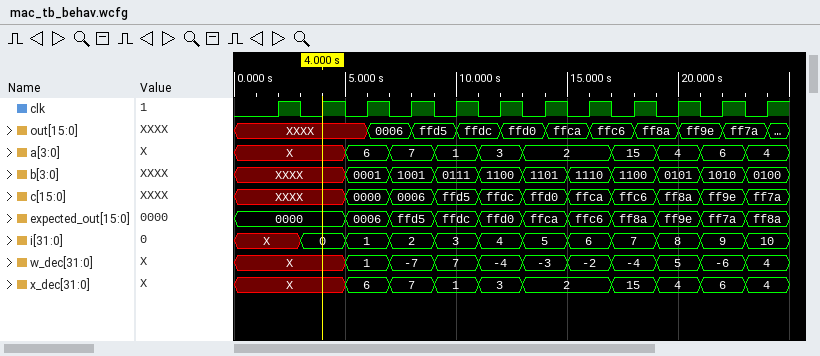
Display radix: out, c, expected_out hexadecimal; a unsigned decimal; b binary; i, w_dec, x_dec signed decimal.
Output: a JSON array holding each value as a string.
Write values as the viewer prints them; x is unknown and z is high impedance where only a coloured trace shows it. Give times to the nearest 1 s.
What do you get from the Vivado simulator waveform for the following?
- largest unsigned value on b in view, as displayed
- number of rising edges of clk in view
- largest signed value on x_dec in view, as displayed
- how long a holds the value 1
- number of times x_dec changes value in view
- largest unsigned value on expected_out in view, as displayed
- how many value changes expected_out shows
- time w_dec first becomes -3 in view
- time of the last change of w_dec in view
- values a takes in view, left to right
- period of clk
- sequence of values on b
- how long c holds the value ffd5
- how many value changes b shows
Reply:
["1110", "12", "15", "2 s", "9", "ffdc", "10", "13 s", "23 s", "X, 6, 7, 1, 3, 2, 15, 4, 6, 4", "2 s", "XXXX, 0001, 1001, 0111, 1100, 1101, 1110, 1100, 0101, 1010, 0100", "2 s", "10"]
